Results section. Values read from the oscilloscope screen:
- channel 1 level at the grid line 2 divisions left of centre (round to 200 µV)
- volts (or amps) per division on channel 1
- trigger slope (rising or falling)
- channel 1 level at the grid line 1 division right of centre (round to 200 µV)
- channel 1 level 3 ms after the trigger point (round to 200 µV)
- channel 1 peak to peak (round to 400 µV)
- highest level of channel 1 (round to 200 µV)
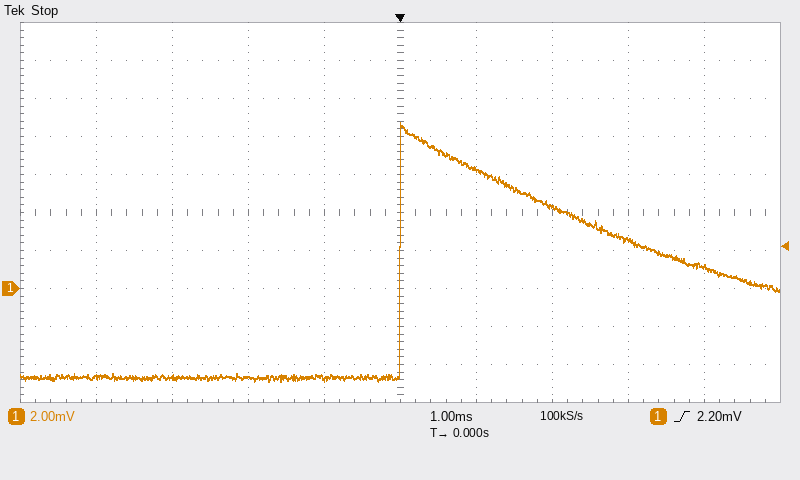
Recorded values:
-4.6 mV
2 mV
rising
6.2 mV
2.6 mV
13.6 mV
8.8 mV
